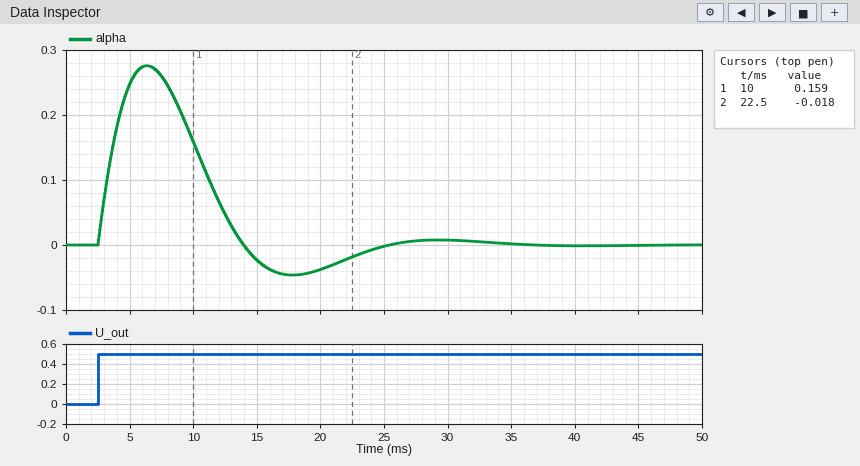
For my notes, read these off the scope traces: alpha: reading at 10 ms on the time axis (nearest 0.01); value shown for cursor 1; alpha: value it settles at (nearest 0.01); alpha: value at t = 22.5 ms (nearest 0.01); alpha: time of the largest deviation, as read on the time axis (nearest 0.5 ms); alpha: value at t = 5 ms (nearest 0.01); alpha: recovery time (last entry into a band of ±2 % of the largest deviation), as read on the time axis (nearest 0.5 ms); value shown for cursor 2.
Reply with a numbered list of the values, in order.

1. 0.16
2. 0.159
3. 0.00
4. -0.02
5. 6.5 ms
6. 0.25
7. 32.0 ms
8. -0.018
